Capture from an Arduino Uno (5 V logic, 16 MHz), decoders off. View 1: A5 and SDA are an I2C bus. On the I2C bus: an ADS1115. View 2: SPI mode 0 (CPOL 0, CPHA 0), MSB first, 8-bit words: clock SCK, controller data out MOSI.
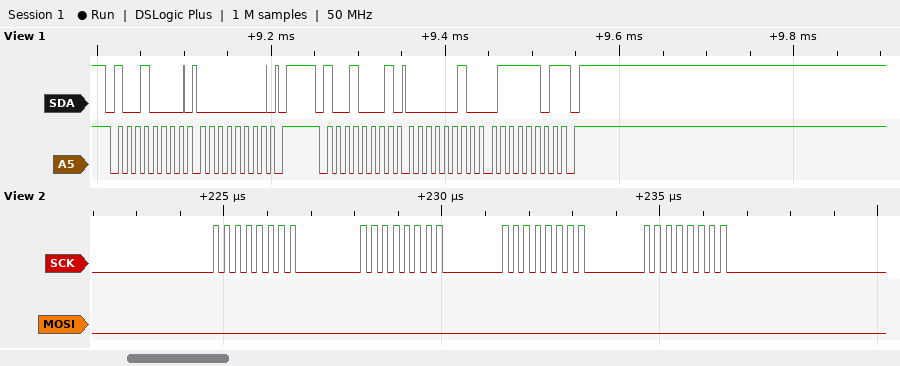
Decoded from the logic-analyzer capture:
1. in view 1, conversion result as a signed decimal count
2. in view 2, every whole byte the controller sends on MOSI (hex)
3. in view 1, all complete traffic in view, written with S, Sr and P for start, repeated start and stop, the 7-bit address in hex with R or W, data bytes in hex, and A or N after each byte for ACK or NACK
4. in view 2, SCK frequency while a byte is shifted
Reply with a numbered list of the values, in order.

1. 637
2. 0x00 0x00 0x00 0x00
3. S 48W A 00 A P S 48R A 02 A 7D N P
4. 4 MHz
